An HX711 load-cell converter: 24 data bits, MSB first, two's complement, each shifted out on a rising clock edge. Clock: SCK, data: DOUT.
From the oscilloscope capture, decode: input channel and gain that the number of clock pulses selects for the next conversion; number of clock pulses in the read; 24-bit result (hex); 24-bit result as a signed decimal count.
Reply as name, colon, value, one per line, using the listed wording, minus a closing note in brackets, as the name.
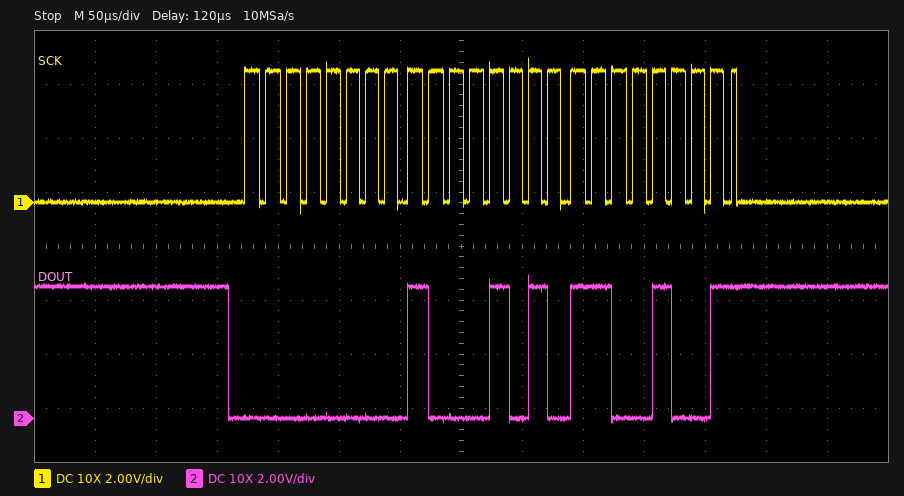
input channel and gain that the number of clock pulses selects for the next conversion: channel A, gain 128
number of clock pulses in the read: 25
24-bit result: 0x008AC9
24-bit result as a signed decimal count: 35529
